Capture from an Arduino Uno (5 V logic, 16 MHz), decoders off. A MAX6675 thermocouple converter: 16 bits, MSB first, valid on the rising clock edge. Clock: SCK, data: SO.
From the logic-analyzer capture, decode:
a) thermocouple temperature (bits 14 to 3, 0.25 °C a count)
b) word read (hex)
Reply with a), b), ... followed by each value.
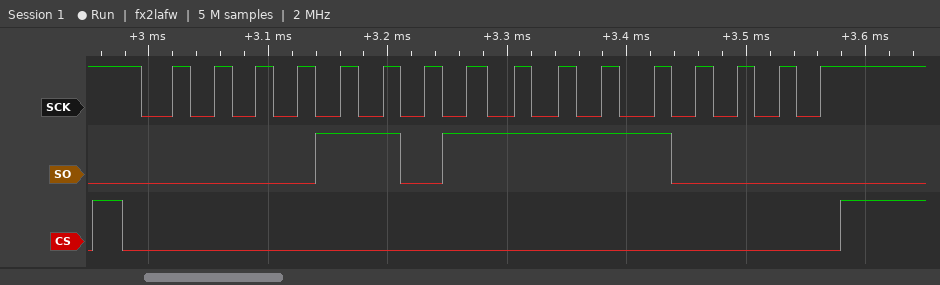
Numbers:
a) 111.50 °C
b) 0x0DF0
